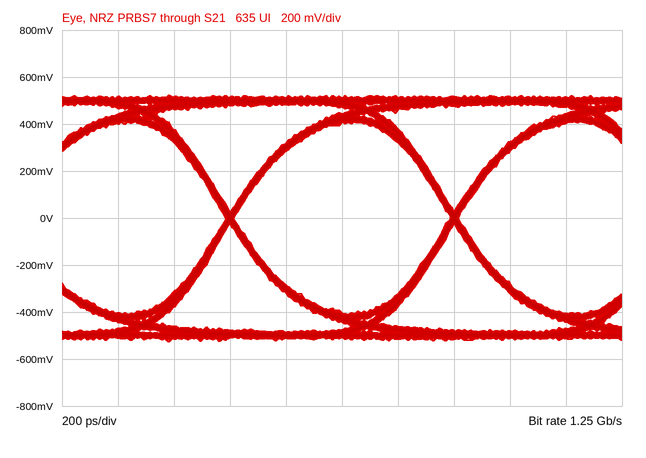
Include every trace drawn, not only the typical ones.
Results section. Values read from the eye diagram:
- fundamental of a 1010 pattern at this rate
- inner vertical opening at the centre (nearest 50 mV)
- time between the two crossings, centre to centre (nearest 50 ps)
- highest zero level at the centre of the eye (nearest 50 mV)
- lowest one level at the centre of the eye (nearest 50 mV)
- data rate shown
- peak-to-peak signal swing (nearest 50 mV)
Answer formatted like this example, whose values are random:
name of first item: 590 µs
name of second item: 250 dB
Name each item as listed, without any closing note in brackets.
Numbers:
fundamental of a 1010 pattern at this rate: 625 MHz
inner vertical opening at the centre: 800 mV
time between the two crossings, centre to centre: 800 ps
highest zero level at the centre of the eye: -400 mV
lowest one level at the centre of the eye: 400 mV
data rate shown: 1.25 Gb/s
peak-to-peak signal swing: 1.05 V
